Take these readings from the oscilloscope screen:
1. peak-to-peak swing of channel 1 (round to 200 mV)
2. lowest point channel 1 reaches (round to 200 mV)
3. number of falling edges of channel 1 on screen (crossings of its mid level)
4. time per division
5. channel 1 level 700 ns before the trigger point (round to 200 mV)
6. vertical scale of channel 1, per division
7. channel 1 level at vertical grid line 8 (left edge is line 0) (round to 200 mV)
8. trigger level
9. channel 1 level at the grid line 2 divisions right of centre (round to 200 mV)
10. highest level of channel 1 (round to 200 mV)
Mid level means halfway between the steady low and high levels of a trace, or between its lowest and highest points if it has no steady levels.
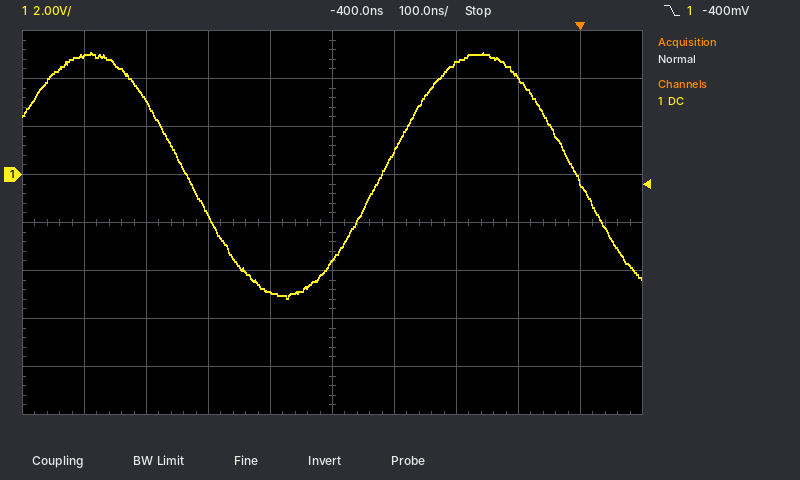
10.2 V
-5.2 V
2
100 ns
3.0 V
2 V
4.0 V
-400 mV
4.6 V
5.0 V
